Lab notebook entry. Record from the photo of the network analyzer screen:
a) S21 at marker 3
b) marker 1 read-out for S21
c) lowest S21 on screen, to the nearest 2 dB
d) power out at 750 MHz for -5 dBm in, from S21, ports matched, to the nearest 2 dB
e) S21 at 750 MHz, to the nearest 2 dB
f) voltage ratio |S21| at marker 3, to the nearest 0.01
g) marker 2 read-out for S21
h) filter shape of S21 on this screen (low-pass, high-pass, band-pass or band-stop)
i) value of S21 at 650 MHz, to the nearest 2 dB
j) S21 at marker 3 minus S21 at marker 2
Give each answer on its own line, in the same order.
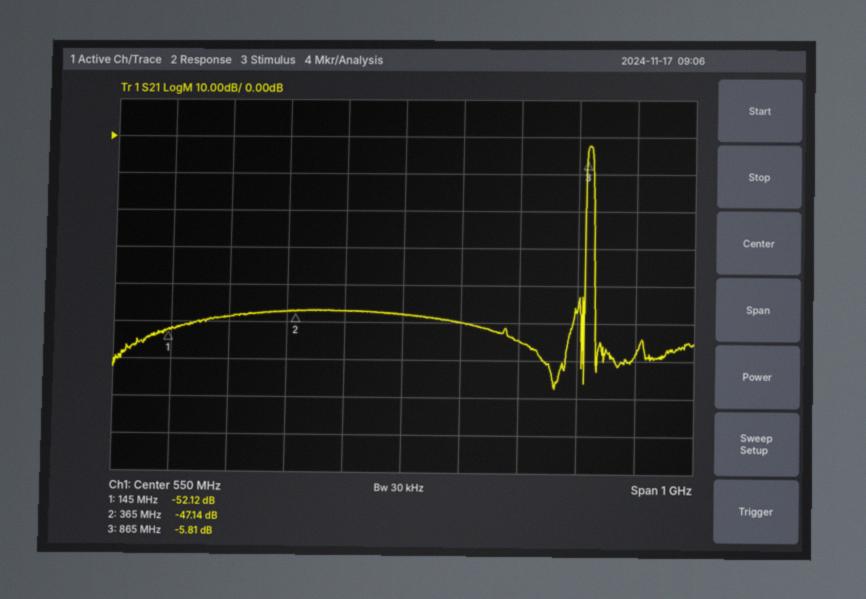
-5.81 dB
-52.12 dB
-68 dB
-60 dBm
-54 dB
0.51
-47.14 dB
band-pass
-50 dB
41.33 dB
